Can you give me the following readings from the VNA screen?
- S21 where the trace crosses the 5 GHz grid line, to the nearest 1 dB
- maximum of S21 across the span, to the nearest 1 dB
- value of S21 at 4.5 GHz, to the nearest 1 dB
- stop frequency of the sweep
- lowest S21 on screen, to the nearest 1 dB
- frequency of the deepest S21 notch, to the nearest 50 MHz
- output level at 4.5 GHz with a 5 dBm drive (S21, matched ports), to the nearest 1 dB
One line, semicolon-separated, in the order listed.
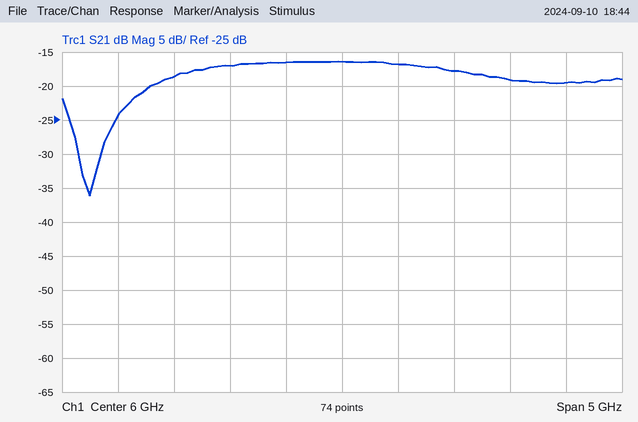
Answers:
-17 dB; -16 dB; -19 dB; 8.5 GHz; -36 dB; 3.75 GHz; -14 dBm
